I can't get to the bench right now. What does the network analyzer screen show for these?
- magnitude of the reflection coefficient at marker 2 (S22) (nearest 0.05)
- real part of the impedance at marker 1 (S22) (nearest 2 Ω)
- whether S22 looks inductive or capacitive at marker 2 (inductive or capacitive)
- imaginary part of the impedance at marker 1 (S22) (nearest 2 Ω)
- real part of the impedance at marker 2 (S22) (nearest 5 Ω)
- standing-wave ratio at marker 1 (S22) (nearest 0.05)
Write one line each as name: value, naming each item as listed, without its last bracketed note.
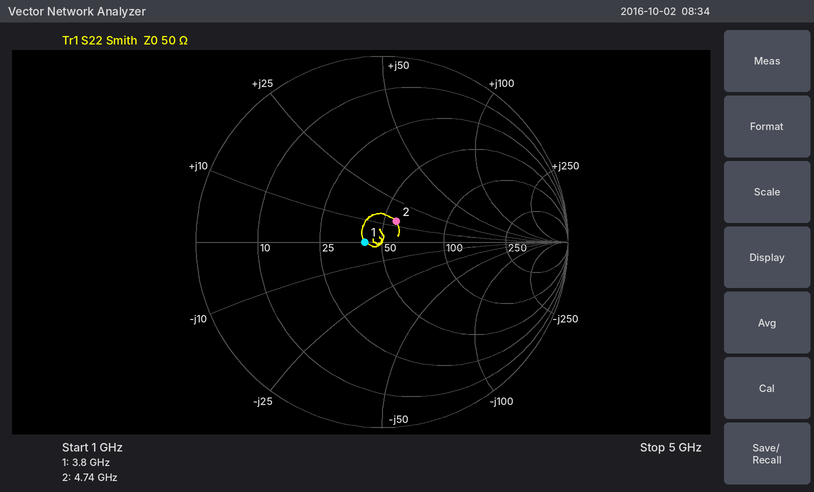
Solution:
magnitude of the reflection coefficient at marker 2 (S22): 0.15
real part of the impedance at marker 1 (S22): 42 Ω
whether S22 looks inductive or capacitive at marker 2: inductive
imaginary part of the impedance at marker 1 (S22): 0 Ω
real part of the impedance at marker 2 (S22): 55 Ω
standing-wave ratio at marker 1 (S22): 1.20
